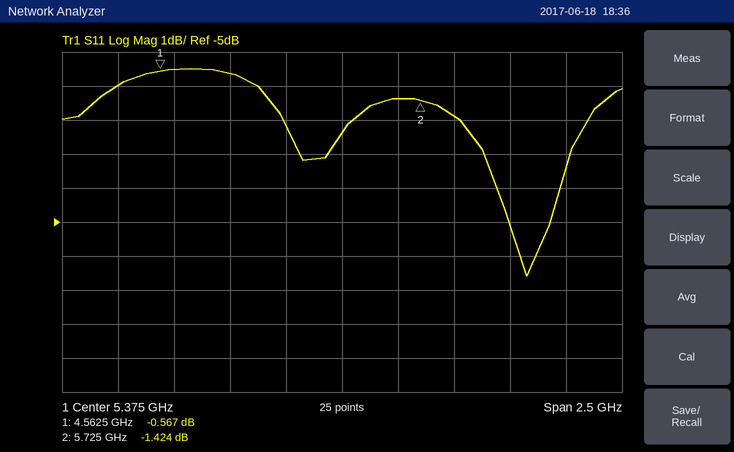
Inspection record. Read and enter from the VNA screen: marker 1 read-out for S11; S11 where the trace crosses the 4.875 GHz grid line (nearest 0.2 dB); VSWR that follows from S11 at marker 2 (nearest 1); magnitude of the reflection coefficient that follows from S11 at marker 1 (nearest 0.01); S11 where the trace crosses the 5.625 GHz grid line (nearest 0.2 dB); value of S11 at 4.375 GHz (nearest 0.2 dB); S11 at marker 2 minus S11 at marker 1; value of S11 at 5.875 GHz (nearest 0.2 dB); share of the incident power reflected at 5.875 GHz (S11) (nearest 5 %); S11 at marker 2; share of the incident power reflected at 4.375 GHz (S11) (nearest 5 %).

-0.567 dB
-0.6 dB
12
0.94
-1.4 dB
-1.0 dB
-0.857 dB
-1.8 dB
65 %
-1.424 dB
80 %
